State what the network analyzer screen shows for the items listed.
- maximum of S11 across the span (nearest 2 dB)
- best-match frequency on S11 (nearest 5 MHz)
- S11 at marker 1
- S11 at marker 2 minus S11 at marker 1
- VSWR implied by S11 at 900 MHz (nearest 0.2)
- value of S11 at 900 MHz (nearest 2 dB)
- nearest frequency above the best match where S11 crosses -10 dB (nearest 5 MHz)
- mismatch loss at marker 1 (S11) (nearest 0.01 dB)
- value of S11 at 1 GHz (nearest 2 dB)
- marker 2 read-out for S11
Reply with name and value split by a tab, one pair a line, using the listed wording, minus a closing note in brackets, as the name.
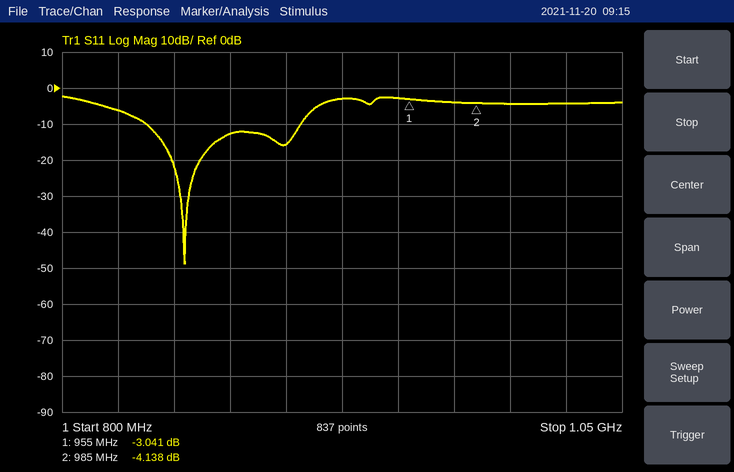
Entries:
maximum of S11 across the span	-2 dB
best-match frequency on S11	855 MHz
S11 at marker 1	-3.041 dB
S11 at marker 2 minus S11 at marker 1	-1.097 dB
VSWR implied by S11 at 900 MHz	1.4
value of S11 at 900 MHz	-16 dB
nearest frequency above the best match where S11 crosses -10 dB	905 MHz
mismatch loss at marker 1 (S11)	2.98 dB
value of S11 at 1 GHz	-4 dB
marker 2 read-out for S11	-4.138 dB
